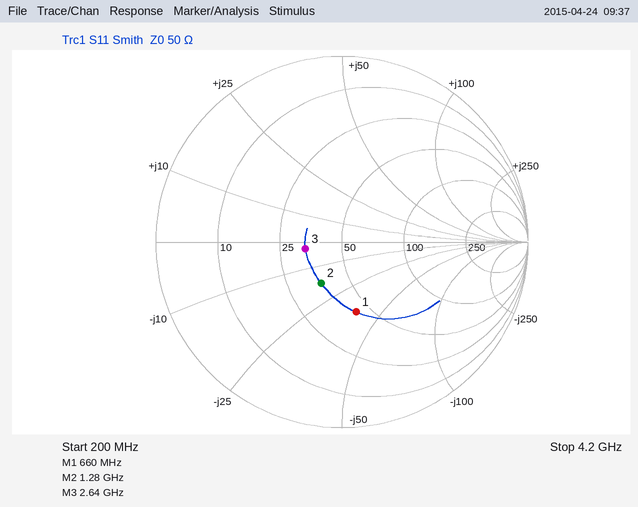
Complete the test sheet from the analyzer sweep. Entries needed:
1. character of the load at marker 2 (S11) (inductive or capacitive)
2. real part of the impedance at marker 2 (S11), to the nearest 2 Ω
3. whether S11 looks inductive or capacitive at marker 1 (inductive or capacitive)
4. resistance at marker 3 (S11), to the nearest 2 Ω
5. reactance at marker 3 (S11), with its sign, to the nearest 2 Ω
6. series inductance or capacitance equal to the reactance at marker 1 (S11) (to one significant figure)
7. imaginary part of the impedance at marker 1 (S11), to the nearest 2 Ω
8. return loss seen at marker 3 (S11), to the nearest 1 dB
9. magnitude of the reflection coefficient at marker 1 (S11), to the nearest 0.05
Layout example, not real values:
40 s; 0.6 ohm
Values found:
capacitive; 36 Ω; capacitive; 34 Ω; -2 Ω; 6 pF; -38 Ω; 14 dB; 0.40
